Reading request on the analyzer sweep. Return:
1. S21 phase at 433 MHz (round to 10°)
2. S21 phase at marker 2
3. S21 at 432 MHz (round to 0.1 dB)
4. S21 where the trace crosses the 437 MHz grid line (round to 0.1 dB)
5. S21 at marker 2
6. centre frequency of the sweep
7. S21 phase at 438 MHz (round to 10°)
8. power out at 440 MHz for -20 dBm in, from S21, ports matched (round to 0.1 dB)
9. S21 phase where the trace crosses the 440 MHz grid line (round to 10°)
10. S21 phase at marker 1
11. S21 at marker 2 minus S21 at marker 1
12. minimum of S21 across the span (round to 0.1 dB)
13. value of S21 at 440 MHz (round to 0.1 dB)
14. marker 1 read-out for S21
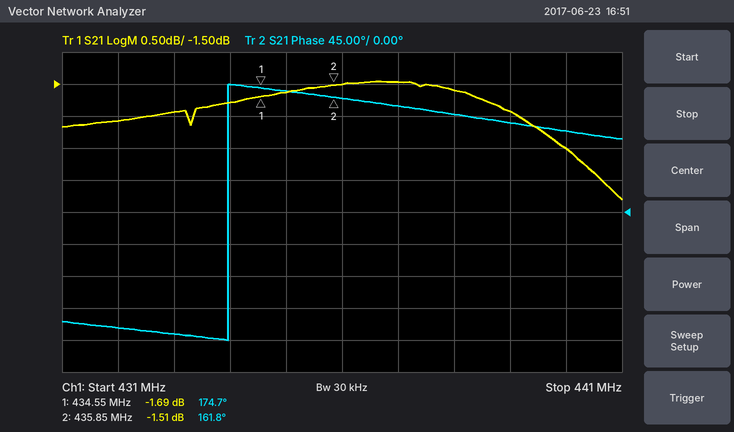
-170°
161.8°
-2.1 dB
-1.5 dB
-1.51 dB
436 MHz
140°
-22.5 dBm
110°
174.7°
0.18 dB
-3.3 dB
-2.5 dB
-1.69 dB
